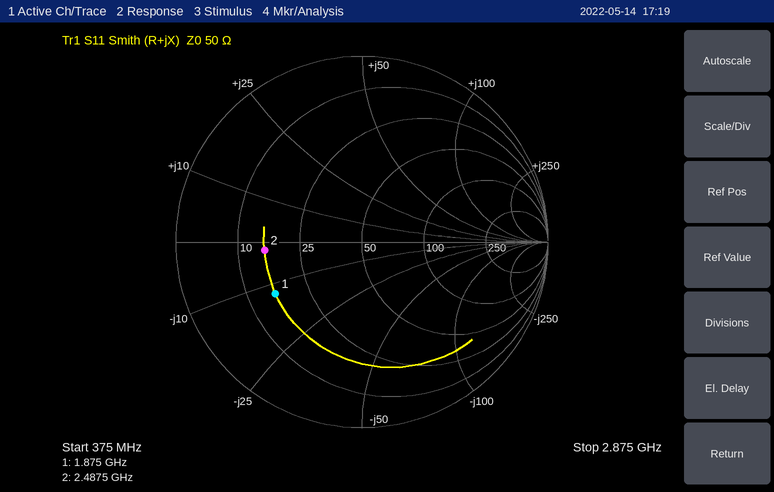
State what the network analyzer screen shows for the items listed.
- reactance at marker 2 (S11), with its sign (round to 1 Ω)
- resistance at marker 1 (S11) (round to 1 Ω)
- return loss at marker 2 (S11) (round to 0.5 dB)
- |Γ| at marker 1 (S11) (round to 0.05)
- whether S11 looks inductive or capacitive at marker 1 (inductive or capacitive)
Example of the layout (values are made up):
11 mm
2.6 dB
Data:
-2 Ω
16 Ω
5.5 dB
0.55
capacitive
